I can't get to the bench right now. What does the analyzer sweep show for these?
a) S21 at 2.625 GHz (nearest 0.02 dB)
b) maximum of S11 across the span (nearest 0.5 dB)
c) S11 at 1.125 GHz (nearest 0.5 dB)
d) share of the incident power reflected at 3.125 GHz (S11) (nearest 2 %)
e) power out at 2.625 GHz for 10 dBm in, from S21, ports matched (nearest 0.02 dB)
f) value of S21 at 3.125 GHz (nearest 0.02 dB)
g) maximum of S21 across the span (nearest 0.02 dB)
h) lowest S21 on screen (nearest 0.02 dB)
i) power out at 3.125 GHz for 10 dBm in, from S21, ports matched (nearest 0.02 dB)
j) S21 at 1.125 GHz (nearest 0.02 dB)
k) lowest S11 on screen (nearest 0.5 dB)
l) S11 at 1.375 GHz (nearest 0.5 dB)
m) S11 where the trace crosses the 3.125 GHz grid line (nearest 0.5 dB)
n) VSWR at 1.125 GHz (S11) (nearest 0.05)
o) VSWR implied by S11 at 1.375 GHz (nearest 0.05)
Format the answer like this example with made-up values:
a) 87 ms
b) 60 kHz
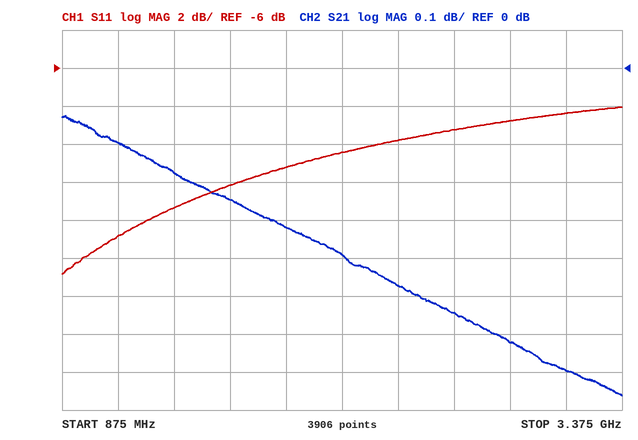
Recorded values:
a) -0.64 dB
b) -8.0 dB
c) -15.0 dB
d) 14 %
e) 9.36 dBm
f) -0.80 dB
g) -0.12 dB
h) -0.86 dB
i) 9.20 dBm
j) -0.20 dB
k) -17.0 dB
l) -13.5 dB
m) -8.5 dB
n) 1.45
o) 1.55
